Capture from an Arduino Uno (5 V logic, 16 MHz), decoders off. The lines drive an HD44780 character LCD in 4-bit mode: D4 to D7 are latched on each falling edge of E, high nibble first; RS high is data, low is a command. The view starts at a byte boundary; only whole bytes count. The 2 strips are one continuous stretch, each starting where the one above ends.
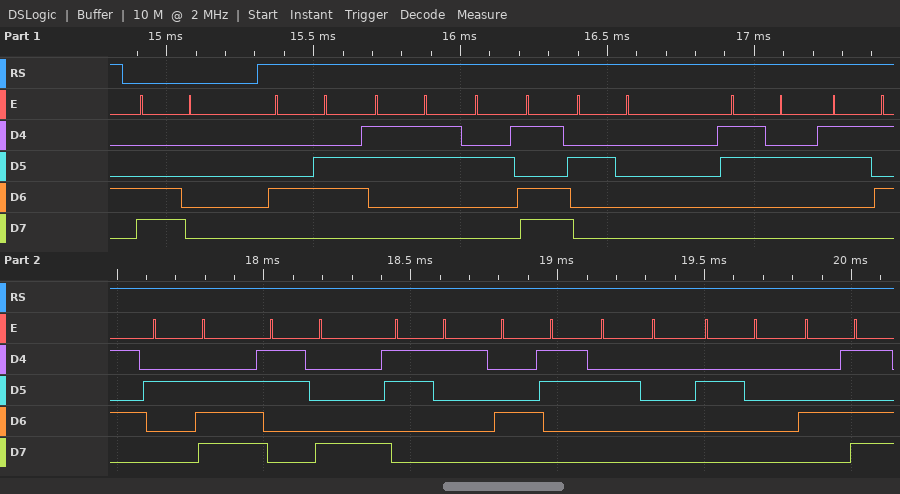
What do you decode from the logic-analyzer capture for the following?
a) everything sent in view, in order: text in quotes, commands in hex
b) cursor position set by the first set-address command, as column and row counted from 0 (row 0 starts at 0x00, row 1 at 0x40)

0xC0 "F3- 25.81C  M"
column 0, row 1
